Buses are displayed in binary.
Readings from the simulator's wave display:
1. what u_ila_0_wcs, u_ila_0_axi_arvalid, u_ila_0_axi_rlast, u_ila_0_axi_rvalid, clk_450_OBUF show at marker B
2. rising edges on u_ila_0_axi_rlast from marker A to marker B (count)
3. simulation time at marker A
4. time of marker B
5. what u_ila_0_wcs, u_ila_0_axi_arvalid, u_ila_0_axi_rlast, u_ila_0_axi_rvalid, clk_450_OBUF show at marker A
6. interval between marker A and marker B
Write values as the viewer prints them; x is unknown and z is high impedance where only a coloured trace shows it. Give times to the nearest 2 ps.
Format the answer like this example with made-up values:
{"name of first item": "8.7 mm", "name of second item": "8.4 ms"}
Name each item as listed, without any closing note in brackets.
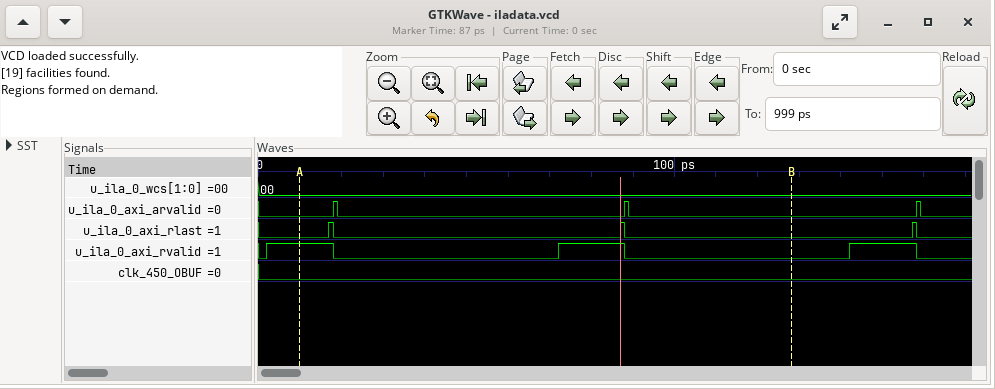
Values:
{"what u_ila_0_wcs, u_ila_0_axi_arvalid, u_ila_0_axi_rlast, u_ila_0_axi_rvalid, clk_450_OBUF show at marker B": "u_ila_0_wcs=00, u_ila_0_axi_arvalid=0, u_ila_0_axi_rlast=0, u_ila_0_axi_rvalid=0, clk_450_OBUF=0", "rising edges on u_ila_0_axi_rlast from marker A to marker B": "2", "simulation time at marker A": "10 ps", "time of marker B": "128 ps", "what u_ila_0_wcs, u_ila_0_axi_arvalid, u_ila_0_axi_rlast, u_ila_0_axi_rvalid, clk_450_OBUF show at marker A": "u_ila_0_wcs=00, u_ila_0_axi_arvalid=0, u_ila_0_axi_rlast=0, u_ila_0_axi_rvalid=1, clk_450_OBUF=0", "interval between marker A and marker B": "118 ps"}
